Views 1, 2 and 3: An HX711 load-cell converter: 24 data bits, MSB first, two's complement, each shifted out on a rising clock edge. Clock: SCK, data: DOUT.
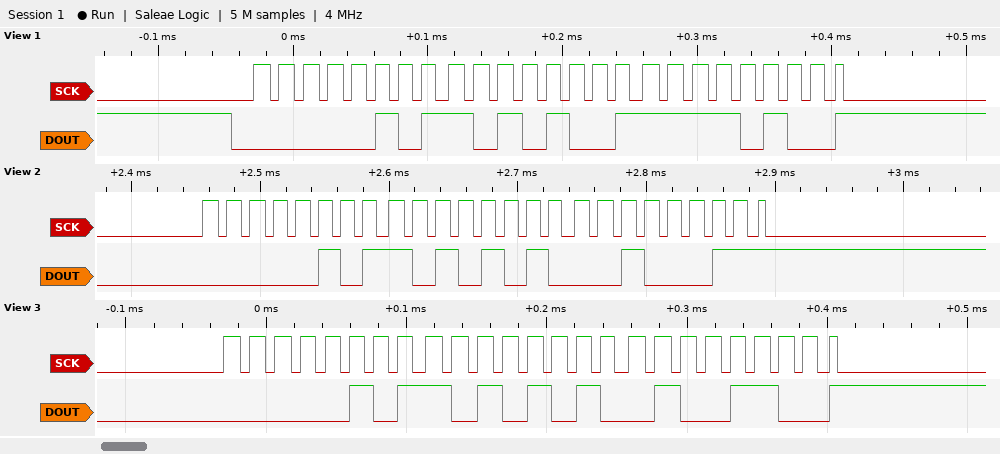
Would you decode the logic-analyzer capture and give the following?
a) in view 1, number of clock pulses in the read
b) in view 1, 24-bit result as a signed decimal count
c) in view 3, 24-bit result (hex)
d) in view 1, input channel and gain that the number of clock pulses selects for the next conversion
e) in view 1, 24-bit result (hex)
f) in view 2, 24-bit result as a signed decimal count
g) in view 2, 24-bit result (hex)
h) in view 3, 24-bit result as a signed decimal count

25
371188
0x05AA4C
channel A, gain 128
0x05A9F4
371235
0x05AA23
371276
